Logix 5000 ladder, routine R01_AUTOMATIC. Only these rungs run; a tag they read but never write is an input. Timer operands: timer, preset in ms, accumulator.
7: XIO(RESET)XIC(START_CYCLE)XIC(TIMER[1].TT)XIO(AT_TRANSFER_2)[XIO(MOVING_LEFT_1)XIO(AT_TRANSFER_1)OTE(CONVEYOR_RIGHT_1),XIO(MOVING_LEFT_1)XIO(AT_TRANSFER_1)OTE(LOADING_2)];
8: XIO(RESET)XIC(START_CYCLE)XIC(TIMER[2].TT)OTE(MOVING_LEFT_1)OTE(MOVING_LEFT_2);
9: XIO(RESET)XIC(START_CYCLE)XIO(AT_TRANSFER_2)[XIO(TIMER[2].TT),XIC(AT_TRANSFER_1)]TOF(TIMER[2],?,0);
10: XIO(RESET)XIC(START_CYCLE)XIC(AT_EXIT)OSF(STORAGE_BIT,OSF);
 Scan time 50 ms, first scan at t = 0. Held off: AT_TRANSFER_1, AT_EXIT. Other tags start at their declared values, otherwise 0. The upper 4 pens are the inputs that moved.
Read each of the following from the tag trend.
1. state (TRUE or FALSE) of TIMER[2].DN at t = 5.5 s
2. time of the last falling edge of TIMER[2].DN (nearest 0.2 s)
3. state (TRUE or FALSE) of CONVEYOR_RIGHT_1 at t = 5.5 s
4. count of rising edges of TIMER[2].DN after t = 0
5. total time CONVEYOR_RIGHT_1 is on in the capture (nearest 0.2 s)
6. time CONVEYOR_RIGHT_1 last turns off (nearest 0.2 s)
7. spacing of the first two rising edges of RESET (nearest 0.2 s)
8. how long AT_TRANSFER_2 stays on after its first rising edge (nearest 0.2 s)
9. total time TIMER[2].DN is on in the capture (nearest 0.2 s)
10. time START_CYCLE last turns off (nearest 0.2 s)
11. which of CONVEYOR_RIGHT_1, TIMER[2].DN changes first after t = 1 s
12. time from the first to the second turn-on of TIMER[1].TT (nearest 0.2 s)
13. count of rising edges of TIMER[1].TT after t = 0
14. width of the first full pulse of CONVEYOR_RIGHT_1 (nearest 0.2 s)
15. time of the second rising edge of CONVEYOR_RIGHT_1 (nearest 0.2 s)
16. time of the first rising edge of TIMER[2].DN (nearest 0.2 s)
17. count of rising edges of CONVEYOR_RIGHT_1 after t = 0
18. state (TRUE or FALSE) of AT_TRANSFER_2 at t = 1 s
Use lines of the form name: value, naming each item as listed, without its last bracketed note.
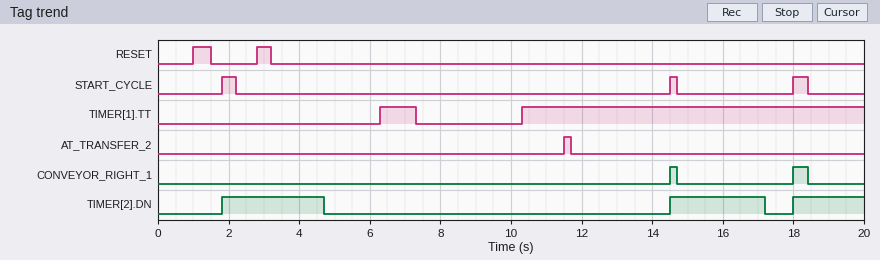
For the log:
state (TRUE or FALSE) of TIMER[2].DN at t = 5.5 s: FALSE
time of the last falling edge of TIMER[2].DN: 17.2 s
state (TRUE or FALSE) of CONVEYOR_RIGHT_1 at t = 5.5 s: FALSE
count of rising edges of TIMER[2].DN after t = 0: 3
total time CONVEYOR_RIGHT_1 is on in the capture: 0.6 s
time CONVEYOR_RIGHT_1 last turns off: 18.4 s
spacing of the first two rising edges of RESET: 1.8 s
how long AT_TRANSFER_2 stays on after its first rising edge: 0.2 s
total time TIMER[2].DN is on in the capture: 7.6 s
time START_CYCLE last turns off: 18.4 s
which of CONVEYOR_RIGHT_1, TIMER[2].DN changes first after t = 1 s: TIMER[2].DN
time from the first to the second turn-on of TIMER[1].TT: 4.0 s
count of rising edges of TIMER[1].TT after t = 0: 2
width of the first full pulse of CONVEYOR_RIGHT_1: 0.2 s
time of the second rising edge of CONVEYOR_RIGHT_1: 18.0 s
time of the first rising edge of TIMER[2].DN: 1.8 s
count of rising edges of CONVEYOR_RIGHT_1 after t = 0: 2
state (TRUE or FALSE) of AT_TRANSFER_2 at t = 1 s: FALSE
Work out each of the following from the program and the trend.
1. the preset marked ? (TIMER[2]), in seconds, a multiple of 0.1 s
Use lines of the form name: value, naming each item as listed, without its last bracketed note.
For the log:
the preset marked ? (TIMER[2]), in seconds, a multiple of 0.1 s: 2.5 s
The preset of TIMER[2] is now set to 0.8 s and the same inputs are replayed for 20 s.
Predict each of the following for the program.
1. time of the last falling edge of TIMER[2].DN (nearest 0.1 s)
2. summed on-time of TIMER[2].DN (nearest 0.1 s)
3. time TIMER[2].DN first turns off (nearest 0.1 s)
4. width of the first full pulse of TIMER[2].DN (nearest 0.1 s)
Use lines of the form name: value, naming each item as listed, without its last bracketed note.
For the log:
time of the last falling edge of TIMER[2].DN: 19.2 s
summed on-time of TIMER[2].DN: 3.4 s
time TIMER[2].DN first turns off: 3.0 s
width of the first full pulse of TIMER[2].DN: 1.2 s
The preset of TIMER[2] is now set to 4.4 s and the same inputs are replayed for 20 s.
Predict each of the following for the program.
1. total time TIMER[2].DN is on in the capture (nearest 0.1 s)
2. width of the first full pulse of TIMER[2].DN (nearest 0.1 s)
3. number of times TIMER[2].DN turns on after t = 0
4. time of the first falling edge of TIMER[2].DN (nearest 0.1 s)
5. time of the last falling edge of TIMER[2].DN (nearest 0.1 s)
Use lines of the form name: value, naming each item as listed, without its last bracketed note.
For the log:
total time TIMER[2].DN is on in the capture: 9.4 s
width of the first full pulse of TIMER[2].DN: 4.8 s
number of times TIMER[2].DN turns on after t = 0: 2
time of the first falling edge of TIMER[2].DN: 6.6 s
time of the last falling edge of TIMER[2].DN: 19.1 s
